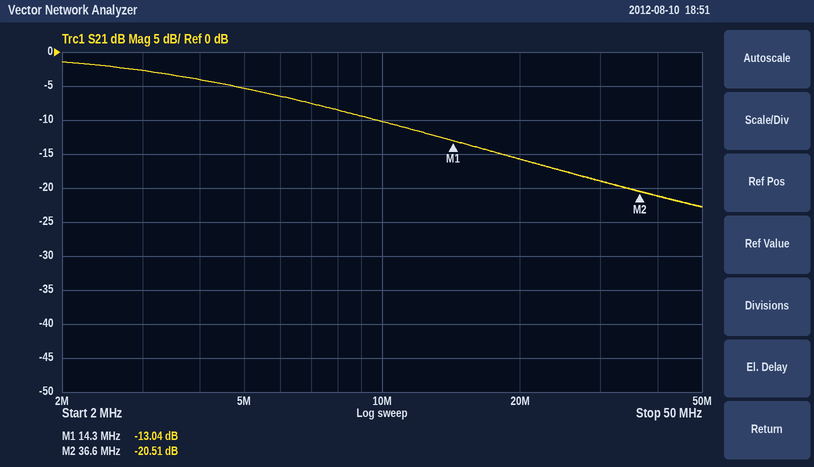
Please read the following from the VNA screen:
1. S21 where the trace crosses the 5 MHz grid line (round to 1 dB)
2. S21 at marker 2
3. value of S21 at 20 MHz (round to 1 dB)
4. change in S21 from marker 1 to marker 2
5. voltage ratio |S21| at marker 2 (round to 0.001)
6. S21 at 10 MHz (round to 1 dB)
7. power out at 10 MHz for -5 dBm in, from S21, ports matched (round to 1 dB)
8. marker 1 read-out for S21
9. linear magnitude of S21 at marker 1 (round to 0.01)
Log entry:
-5 dB
-20.51 dB
-16 dB
-7.47 dB
0.094
-10 dB
-15 dBm
-13.04 dB
0.22
